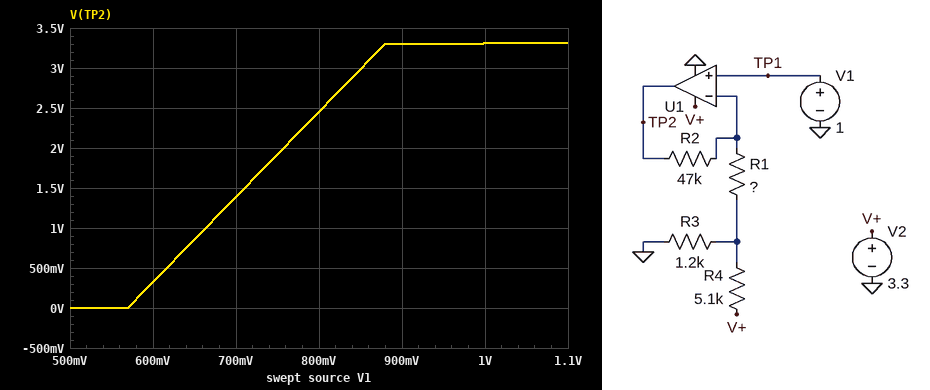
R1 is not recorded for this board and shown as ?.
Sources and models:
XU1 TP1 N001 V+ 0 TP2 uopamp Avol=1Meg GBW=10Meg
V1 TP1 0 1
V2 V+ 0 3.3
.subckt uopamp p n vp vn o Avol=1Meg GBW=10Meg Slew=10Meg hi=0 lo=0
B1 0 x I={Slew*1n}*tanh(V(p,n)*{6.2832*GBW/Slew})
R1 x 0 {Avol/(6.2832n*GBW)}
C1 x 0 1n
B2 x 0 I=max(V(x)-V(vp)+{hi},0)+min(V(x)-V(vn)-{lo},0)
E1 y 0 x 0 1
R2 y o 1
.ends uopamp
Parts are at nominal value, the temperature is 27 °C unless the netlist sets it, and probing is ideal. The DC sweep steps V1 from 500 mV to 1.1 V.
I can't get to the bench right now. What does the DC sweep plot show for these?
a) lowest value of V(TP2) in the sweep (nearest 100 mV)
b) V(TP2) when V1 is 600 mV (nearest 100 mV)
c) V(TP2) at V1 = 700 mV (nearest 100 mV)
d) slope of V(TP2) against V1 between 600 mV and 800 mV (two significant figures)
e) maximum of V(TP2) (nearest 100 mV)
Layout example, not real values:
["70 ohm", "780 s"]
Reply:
["0 V", "300 mV", "1.4 V", "11 V/V", "3.3 V"]
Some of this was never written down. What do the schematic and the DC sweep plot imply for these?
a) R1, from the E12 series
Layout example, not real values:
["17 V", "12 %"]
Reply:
["3.9 kΩ"]
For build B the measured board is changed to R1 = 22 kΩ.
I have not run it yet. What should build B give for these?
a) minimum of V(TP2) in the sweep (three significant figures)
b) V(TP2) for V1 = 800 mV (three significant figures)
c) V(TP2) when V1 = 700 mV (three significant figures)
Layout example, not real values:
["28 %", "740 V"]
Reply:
["237 mV", "1.15 V", "846 mV"]
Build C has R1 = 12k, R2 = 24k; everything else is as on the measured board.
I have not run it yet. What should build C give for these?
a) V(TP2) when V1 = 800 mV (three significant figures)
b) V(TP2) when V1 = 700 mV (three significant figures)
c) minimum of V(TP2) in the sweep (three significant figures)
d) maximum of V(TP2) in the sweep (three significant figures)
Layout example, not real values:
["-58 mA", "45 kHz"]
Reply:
["1.12 V", "832 mV", "262 mV", "1.97 V"]
